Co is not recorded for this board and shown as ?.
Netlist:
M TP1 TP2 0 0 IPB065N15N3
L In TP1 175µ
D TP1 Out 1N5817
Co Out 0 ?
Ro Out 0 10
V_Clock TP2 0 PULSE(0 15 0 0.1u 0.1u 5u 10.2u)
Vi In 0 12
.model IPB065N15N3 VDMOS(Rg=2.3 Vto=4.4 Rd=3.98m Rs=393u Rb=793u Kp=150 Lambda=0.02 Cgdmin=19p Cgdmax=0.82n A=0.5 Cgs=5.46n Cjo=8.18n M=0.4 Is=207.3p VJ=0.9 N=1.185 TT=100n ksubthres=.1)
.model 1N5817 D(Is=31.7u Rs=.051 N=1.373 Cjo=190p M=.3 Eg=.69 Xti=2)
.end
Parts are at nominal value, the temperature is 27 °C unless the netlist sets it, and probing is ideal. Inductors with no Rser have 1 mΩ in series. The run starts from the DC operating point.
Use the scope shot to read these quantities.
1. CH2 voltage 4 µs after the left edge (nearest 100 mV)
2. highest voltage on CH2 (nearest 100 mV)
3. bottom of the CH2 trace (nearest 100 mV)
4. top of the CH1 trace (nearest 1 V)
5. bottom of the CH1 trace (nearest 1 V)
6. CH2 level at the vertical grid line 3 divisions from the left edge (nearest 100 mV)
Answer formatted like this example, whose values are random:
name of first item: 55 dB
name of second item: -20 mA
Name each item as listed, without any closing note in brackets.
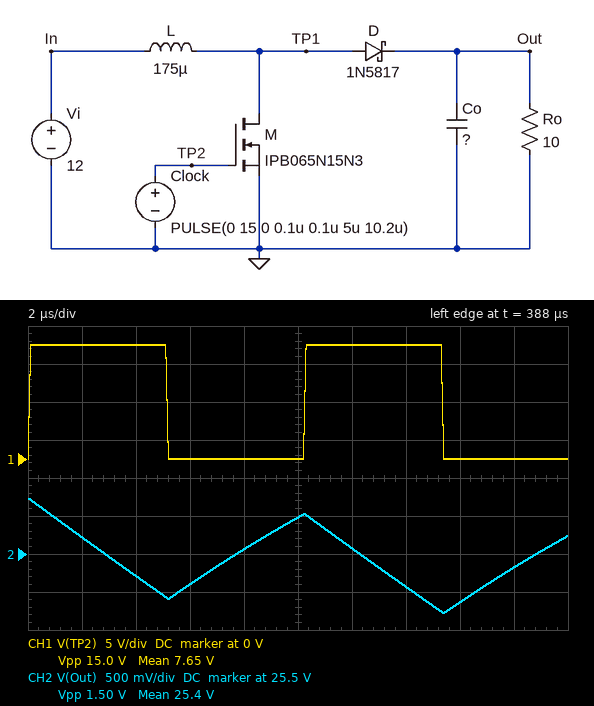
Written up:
CH2 voltage 4 µs after the left edge: 25.2 V
highest voltage on CH2: 26.2 V
bottom of the CH2 trace: 24.7 V
top of the CH1 trace: 15 V
bottom of the CH1 trace: 0 V
CH2 level at the vertical grid line 3 divisions from the left edge: 25.1 V
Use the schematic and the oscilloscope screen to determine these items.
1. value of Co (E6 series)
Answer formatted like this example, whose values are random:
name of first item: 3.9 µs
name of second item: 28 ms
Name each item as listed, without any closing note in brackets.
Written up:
value of Co: 10 µF
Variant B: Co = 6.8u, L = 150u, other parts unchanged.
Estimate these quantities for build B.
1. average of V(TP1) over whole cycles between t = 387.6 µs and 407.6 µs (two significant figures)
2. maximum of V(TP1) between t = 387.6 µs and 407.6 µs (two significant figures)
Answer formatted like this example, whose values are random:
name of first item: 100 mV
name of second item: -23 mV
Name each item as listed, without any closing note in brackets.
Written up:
average of V(TP1) over whole cycles between t = 387.6 µs and 407.6 µs: 12 V
maximum of V(TP1) between t = 387.6 µs and 407.6 µs: 25 V
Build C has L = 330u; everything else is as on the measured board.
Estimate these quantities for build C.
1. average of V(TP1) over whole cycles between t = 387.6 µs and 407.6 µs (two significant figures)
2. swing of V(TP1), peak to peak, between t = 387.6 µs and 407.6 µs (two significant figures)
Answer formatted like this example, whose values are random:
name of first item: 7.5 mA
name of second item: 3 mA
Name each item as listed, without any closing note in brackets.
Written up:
average of V(TP1) over whole cycles between t = 387.6 µs and 407.6 µs: 12 V
swing of V(TP1), peak to peak, between t = 387.6 µs and 407.6 µs: 26 V
